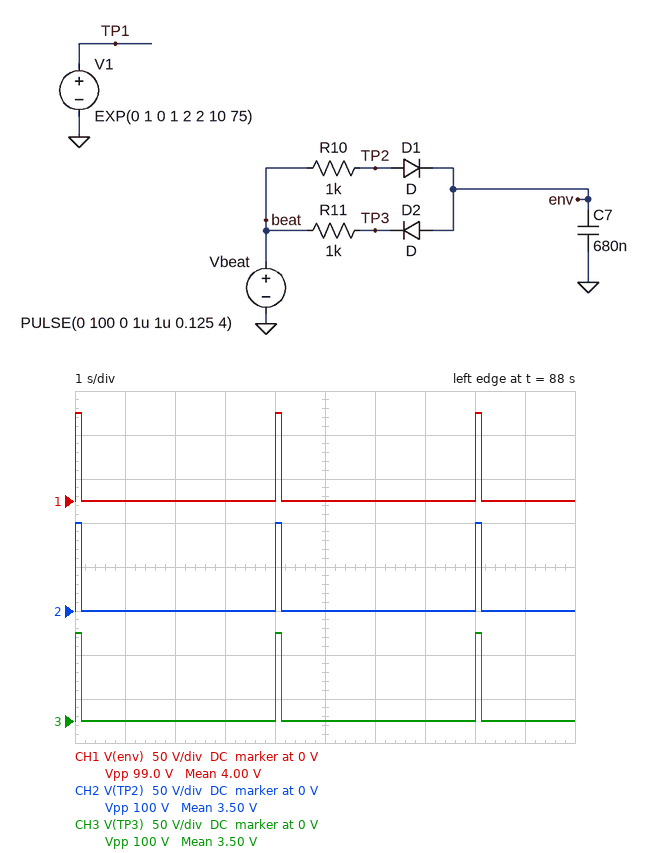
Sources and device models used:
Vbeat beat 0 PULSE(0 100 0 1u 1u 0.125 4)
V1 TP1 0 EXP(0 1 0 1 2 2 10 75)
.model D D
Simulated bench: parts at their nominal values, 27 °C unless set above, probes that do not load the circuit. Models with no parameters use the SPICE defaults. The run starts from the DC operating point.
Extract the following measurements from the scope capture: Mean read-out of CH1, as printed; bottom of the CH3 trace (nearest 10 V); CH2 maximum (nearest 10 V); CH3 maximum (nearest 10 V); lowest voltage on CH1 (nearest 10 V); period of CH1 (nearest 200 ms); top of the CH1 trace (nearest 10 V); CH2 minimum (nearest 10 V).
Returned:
4.00 V
0 V
100 V
100 V
0 V
4.0 s
100 V
0 V
